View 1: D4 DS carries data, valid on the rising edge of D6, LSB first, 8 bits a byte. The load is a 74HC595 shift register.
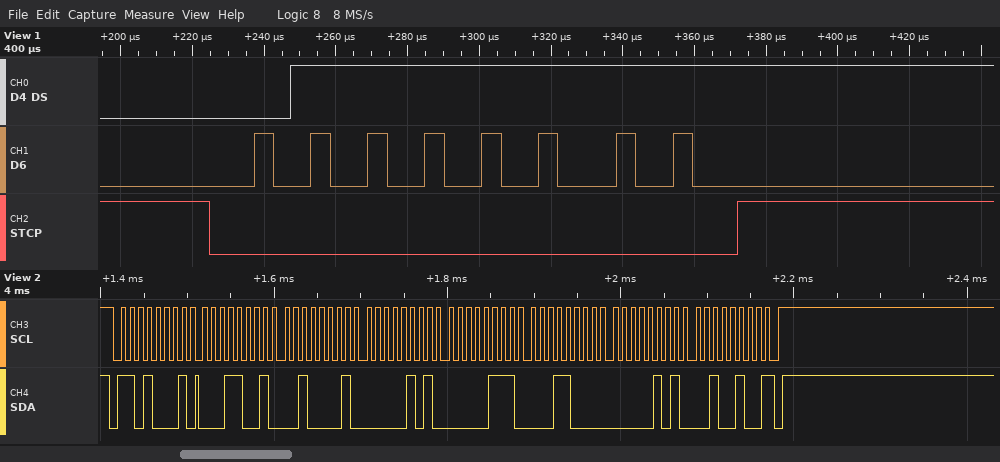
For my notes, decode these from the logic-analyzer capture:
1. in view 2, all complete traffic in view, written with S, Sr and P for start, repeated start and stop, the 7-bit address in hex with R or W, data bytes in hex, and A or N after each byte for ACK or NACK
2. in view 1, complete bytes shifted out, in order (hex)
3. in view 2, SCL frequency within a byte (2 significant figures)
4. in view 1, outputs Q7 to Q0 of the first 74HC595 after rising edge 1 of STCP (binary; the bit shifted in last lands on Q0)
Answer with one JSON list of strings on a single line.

["S 68R A 19 A 21 A 05 A 07 A 18 A 05 A 24 N P", "FE", "100 kHz", "01111111"]
